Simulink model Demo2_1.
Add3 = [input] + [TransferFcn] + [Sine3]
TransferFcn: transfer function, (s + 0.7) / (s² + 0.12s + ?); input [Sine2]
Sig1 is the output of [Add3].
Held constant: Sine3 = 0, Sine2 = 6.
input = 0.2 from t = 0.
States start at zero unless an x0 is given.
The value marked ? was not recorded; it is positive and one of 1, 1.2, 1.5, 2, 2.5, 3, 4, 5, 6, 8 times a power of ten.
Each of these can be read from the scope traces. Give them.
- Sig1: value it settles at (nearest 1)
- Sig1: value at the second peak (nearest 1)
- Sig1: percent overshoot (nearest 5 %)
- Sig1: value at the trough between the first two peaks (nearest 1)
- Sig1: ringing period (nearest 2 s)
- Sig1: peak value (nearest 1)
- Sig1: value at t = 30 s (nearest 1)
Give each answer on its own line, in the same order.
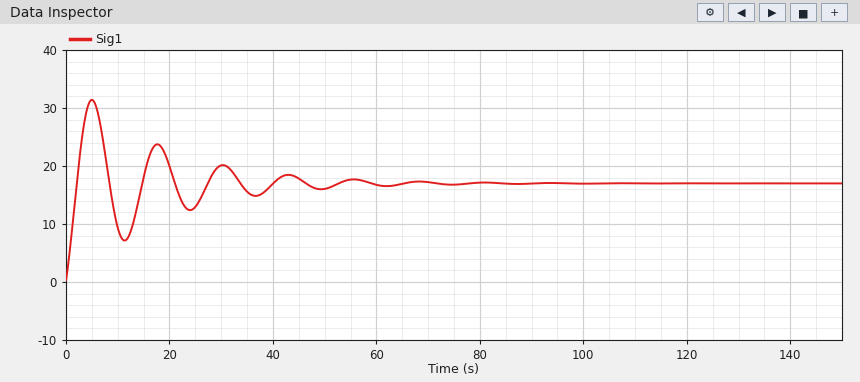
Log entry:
17
24
85 %
7
12 s
31
20
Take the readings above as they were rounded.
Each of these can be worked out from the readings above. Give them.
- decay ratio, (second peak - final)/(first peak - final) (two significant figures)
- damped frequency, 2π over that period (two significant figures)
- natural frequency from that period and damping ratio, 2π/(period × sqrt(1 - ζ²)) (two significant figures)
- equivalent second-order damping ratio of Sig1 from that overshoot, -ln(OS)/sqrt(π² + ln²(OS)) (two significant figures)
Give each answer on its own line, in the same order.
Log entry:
0.50
0.52 rad/s
0.52 rad/s
0.052
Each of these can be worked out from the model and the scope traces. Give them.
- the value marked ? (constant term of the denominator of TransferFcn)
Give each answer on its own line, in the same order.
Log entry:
0.25
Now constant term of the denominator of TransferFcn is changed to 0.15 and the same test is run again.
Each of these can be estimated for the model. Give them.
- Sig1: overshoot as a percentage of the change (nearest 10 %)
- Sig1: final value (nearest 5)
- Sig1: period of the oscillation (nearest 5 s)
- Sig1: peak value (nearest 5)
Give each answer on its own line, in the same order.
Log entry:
70 %
30
15 s
50
